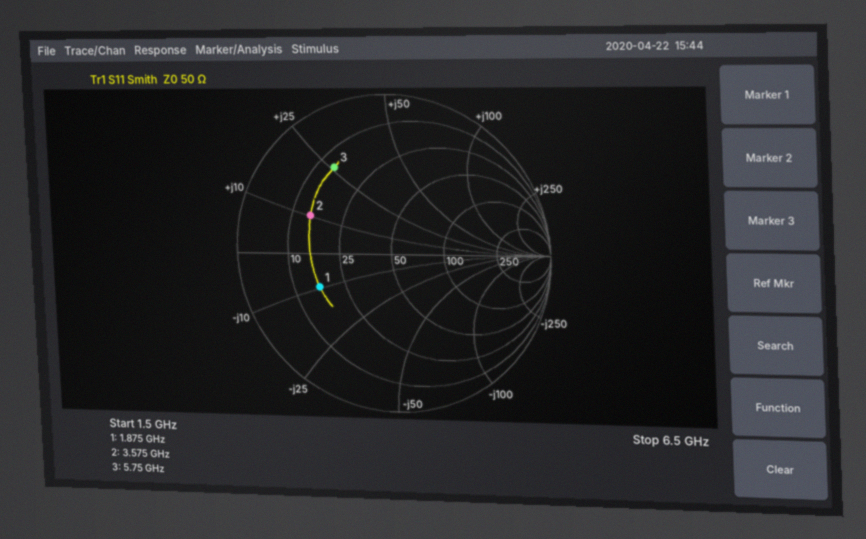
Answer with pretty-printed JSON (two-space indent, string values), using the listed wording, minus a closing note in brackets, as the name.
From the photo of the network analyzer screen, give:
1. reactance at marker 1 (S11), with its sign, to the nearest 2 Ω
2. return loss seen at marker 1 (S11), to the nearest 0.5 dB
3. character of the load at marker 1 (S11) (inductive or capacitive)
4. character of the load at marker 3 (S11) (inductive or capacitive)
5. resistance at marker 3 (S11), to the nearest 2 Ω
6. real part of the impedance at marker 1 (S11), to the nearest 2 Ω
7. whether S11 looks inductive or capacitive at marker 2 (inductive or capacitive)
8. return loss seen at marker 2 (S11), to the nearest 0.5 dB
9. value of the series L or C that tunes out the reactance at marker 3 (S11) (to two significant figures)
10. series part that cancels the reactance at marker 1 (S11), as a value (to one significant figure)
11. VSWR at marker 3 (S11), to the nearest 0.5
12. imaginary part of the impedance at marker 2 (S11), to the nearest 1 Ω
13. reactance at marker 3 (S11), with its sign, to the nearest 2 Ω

{
  "reactance at marker 1 (S11), with its sign, to the nearest 2 Ω": "-10 Ω",
  "return loss seen at marker 1 (S11), to the nearest 0.5 dB": "5.5 dB",
  "character of the load at marker 1 (S11)": "capacitive",
  "character of the load at marker 3 (S11)": "inductive",
  "resistance at marker 3 (S11), to the nearest 2 Ω": "14 Ω",
  "real part of the impedance at marker 1 (S11), to the nearest 2 Ω": "16 Ω",
  "whether S11 looks inductive or capacitive at marker 2": "inductive",
  "return loss seen at marker 2 (S11), to the nearest 0.5 dB": "5.0 dB",
  "value of the series L or C that tunes out the reactance at marker 3 (S11)": "1.1 pF",
  "series part that cancels the reactance at marker 1 (S11), as a value": "800 pH",
  "VSWR at marker 3 (S11), to the nearest 0.5": "4.5",
  "imaginary part of the impedance at marker 2 (S11), to the nearest 1 Ω": "+10 Ω",
  "reactance at marker 3 (S11), with its sign, to the nearest 2 Ω": "+26 Ω"
}
